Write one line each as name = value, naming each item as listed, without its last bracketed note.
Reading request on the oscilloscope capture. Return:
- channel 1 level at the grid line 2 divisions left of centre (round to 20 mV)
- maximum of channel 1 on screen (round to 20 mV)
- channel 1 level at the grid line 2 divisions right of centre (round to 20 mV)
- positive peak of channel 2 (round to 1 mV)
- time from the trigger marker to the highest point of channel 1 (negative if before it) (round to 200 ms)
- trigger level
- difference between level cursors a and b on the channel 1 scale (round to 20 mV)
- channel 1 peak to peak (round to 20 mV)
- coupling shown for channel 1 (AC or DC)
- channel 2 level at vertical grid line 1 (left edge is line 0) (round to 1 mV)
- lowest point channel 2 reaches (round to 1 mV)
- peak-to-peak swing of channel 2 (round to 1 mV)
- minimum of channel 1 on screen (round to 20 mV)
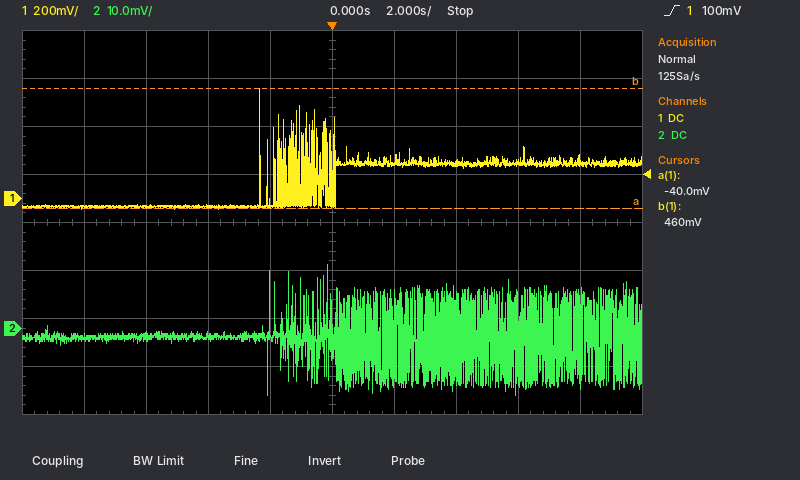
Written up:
channel 1 level at the grid line 2 divisions left of centre = -40 mV
maximum of channel 1 on screen = 460 mV
channel 1 level at the grid line 2 divisions right of centre = 140 mV
positive peak of channel 2 = 13 mV
time from the trigger marker to the highest point of channel 1 (negative if before it) = -2.4 s
trigger level = 100 mV
difference between level cursors a and b on the channel 1 scale = 500 mV
channel 1 peak to peak = 500 mV
coupling shown for channel 1 = DC
channel 2 level at vertical grid line 1 (left edge is line 0) = -2 mV
lowest point channel 2 reaches = -14 mV
peak-to-peak swing of channel 2 = 27 mV
minimum of channel 1 on screen = -40 mV
